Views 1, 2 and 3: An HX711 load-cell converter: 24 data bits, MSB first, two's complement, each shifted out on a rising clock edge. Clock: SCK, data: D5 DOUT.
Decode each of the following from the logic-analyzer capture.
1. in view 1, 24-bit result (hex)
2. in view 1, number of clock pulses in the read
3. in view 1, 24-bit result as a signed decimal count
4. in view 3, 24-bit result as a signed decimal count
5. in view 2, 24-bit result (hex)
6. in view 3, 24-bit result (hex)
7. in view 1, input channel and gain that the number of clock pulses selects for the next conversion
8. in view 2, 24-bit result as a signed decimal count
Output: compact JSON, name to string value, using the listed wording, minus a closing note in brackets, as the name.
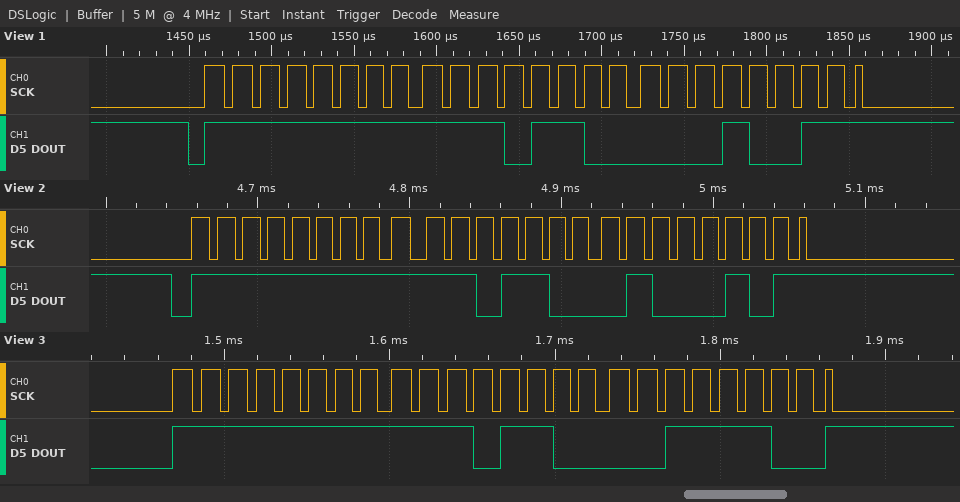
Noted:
{"in view 1, 24-bit result": "0xFFEC13", "in view 1, number of clock pulses in the read": "25", "in view 1, 24-bit result as a signed decimal count": "-5101", "in view 3, 24-bit result as a signed decimal count": "-5060", "in view 2, 24-bit result": "0xFFEC45", "in view 3, 24-bit result": "0xFFEC3C", "in view 1, input channel and gain that the number of clock pulses selects for the next conversion": "channel A, gain 128", "in view 2, 24-bit result as a signed decimal count": "-5051"}
